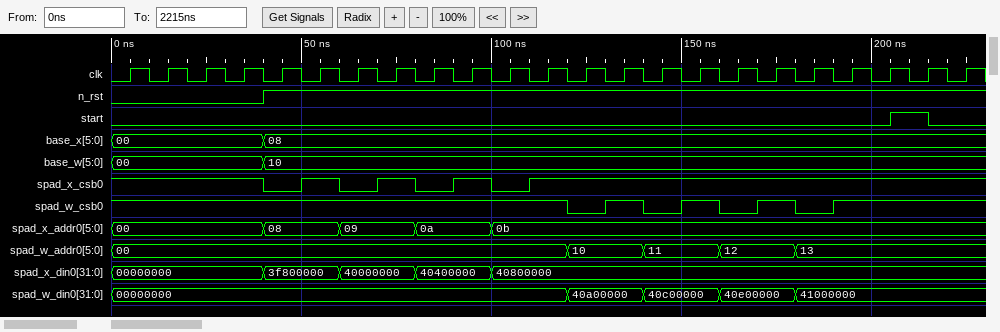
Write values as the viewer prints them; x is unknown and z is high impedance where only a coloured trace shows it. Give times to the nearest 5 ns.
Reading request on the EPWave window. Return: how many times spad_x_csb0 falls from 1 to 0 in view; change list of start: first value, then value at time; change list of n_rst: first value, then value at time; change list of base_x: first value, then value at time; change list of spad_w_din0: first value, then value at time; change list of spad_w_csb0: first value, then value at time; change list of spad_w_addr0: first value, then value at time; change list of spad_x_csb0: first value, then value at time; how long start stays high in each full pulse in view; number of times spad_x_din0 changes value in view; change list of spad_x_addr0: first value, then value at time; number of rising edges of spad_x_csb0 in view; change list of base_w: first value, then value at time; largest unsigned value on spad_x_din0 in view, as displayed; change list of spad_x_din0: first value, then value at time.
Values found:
4
0, 1 at 205 ns, 0 at 215 ns
0, 1 at 40 ns
00, 08 at 40 ns
00000000, 40a00000 at 120 ns, 40c00000 at 140 ns, 40e00000 at 160 ns, 41000000 at 180 ns
1, 0 at 120 ns, 1 at 130 ns, 0 at 140 ns, 1 at 150 ns, 0 at 160 ns, 1 at 170 ns, 0 at 180 ns, 1 at 190 ns
00, 10 at 120 ns, 11 at 140 ns, 12 at 160 ns, 13 at 180 ns
1, 0 at 40 ns, 1 at 50 ns, 0 at 60 ns, 1 at 70 ns, 0 at 80 ns, 1 at 90 ns, 0 at 100 ns, 1 at 110 ns
10 ns
4
00, 08 at 40 ns, 09 at 60 ns, 0a at 80 ns, 0b at 100 ns
4
00, 10 at 40 ns
40800000
00000000, 3f800000 at 40 ns, 40000000 at 60 ns, 40400000 at 80 ns, 40800000 at 100 ns
